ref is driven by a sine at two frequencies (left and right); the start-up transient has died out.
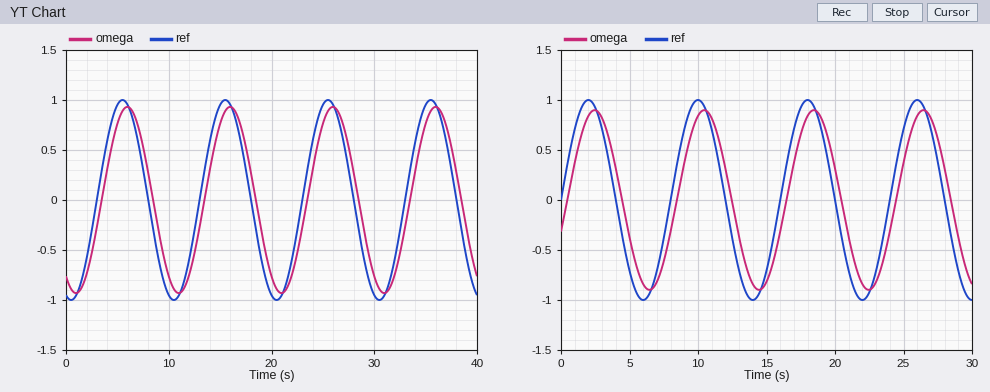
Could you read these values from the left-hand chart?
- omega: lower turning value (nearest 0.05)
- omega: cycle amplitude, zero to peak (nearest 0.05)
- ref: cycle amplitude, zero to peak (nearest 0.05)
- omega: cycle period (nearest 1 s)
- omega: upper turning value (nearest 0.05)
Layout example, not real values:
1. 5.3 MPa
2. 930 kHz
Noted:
1. -0.95
2. 0.95
3. 1.00
4. 10 s
5. 0.95
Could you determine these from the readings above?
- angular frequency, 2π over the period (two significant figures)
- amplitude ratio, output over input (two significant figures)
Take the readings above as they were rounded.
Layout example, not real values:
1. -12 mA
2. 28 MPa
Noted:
1. 0.63 rad/s
2. 0.95
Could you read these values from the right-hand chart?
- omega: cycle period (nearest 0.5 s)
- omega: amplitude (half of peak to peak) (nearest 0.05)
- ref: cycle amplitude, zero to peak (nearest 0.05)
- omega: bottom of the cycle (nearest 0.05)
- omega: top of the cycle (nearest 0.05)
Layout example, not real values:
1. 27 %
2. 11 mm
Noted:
1. 8.0 s
2. 0.90
3. 1.00
4. -0.90
5. 0.90
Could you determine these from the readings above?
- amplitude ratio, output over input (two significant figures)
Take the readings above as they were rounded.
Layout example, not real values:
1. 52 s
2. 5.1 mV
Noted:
1. 0.90
